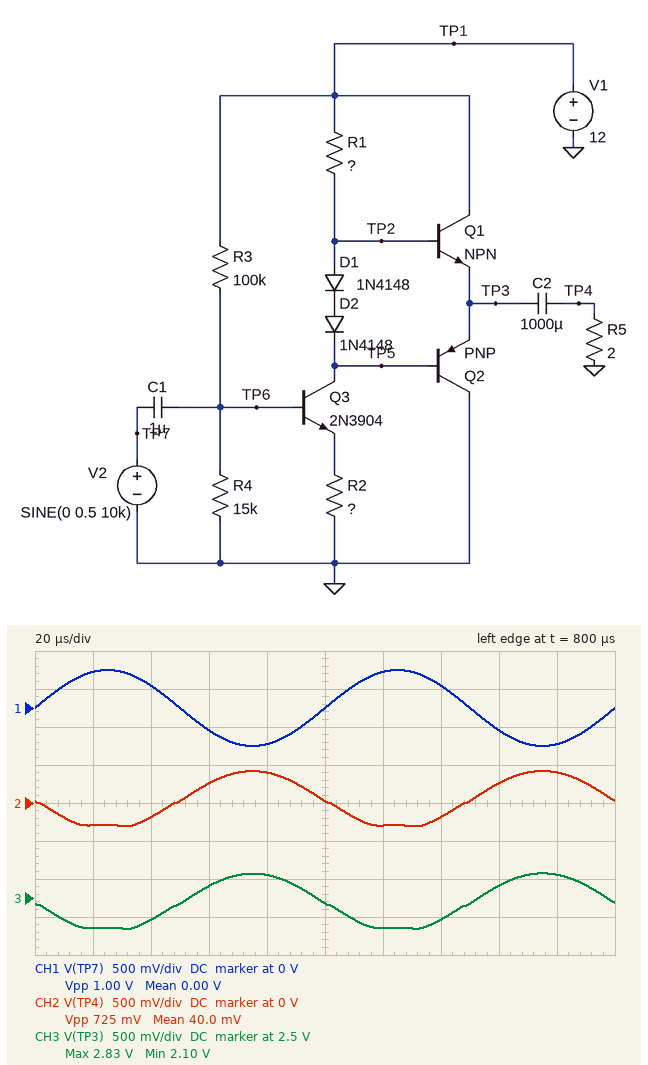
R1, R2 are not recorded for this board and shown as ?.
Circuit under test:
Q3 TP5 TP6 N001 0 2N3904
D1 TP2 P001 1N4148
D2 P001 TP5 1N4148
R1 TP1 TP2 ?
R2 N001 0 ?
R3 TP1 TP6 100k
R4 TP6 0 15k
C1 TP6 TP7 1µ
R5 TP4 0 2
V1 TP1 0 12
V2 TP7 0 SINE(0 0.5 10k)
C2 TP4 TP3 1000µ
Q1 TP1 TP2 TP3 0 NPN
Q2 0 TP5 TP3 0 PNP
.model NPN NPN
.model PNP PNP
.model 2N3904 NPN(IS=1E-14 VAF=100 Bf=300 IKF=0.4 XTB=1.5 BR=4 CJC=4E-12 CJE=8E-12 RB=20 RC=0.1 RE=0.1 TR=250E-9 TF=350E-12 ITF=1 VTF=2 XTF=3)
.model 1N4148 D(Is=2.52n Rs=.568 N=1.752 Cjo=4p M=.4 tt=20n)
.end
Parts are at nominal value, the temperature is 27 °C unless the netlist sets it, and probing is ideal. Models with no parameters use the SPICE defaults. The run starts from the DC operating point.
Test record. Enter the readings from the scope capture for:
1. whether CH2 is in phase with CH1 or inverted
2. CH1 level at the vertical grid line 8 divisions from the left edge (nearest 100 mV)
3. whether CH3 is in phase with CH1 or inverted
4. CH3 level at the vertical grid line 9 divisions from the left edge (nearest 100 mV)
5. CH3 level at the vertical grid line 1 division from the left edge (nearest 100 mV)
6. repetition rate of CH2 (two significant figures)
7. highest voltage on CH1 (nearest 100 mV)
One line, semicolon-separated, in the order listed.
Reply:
inverted; -300 mV; inverted; 2.8 V; 2.1 V; 10 kHz; 500 mV
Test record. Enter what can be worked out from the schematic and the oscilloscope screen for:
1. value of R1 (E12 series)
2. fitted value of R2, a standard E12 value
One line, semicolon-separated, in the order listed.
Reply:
2.7 kΩ; 220 Ω
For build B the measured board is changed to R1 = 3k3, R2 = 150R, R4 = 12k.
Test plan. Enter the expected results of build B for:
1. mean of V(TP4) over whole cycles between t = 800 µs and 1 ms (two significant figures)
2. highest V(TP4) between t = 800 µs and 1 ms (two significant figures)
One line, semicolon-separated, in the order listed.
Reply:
300 mV; 560 mV
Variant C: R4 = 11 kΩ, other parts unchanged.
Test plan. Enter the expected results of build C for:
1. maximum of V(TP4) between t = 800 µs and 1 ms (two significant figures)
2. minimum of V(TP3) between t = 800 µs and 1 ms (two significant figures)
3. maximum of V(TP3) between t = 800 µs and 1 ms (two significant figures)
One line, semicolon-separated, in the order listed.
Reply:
340 mV; 5.5 V; 6.2 V
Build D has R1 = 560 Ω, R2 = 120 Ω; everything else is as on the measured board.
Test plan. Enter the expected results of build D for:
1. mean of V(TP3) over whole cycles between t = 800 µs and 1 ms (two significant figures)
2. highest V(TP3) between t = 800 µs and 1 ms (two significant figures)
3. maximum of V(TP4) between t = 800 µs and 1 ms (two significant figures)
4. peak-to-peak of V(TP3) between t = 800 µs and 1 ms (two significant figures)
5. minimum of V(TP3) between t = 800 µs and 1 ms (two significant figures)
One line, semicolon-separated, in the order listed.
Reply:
8.3 V; 8.8 V; 510 mV; 1.0 V; 7.8 V
